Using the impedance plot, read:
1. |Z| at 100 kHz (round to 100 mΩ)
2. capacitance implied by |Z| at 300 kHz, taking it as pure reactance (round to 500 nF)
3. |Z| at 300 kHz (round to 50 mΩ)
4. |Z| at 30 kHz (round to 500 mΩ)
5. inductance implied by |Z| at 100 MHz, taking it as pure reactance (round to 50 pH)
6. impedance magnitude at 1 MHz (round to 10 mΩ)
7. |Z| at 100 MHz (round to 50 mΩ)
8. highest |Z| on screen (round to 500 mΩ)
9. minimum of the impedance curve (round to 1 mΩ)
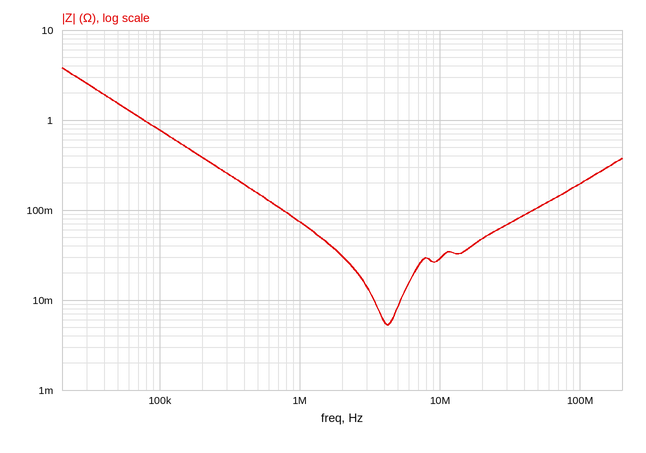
800 mΩ
2.0 µF
250 mΩ
2.5 Ω
300 pH
70 mΩ
200 mΩ
4.0 Ω
5 mΩ
